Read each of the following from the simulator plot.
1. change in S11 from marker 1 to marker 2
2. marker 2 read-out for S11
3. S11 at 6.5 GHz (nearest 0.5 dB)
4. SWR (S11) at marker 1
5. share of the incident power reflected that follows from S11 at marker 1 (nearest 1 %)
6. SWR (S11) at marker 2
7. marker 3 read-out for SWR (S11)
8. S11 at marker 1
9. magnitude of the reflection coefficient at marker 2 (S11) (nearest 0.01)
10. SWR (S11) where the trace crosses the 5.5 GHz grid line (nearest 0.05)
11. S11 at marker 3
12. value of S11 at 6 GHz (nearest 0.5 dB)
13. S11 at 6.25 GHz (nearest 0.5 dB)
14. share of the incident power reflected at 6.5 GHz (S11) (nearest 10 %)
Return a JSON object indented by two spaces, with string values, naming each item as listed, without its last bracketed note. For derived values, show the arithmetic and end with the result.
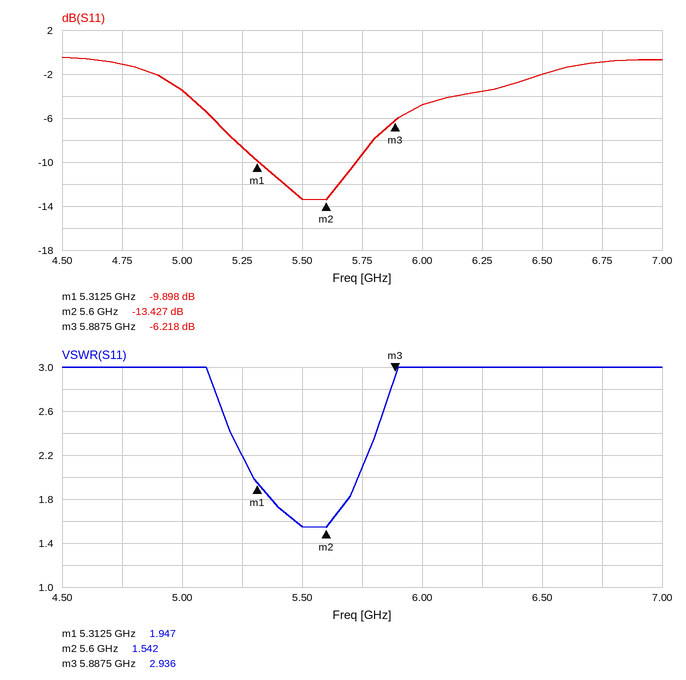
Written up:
{
  "change in S11 from marker 1 to marker 2": "-13.427 − (-9.898) = -3.529 dB",
  "marker 2 read-out for S11": "-13.427 dB",
  "S11 at 6.5 GHz": "-2.0 dB",
  "SWR (S11) at marker 1": "1.947",
  "share of the incident power reflected that follows from S11 at marker 1": "10^(-9.898/10) ≈ 10 %",
  "SWR (S11) at marker 2": "1.542",
  "marker 3 read-out for SWR": "2.936",
  "S11 at marker 1": "-9.898 dB",
  "magnitude of the reflection coefficient at marker 2 (S11)": "10^(-13.427/20) ≈ 0.21",
  "SWR (S11) where the trace crosses the 5.5 GHz grid line": "1.55",
  "S11 at marker 3": "-6.218 dB",
  "value of S11 at 6 GHz": "-5.0 dB",
  "S11 at 6.25 GHz": "-3.5 dB",
  "share of the incident power reflected at 6.5 GHz (S11)": "10^(-2/10) ≈ 63.1 %, so 60 % to the nearest 10 %"
}
